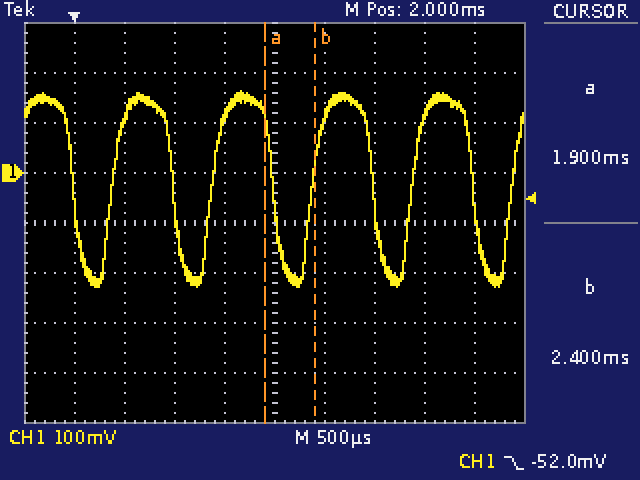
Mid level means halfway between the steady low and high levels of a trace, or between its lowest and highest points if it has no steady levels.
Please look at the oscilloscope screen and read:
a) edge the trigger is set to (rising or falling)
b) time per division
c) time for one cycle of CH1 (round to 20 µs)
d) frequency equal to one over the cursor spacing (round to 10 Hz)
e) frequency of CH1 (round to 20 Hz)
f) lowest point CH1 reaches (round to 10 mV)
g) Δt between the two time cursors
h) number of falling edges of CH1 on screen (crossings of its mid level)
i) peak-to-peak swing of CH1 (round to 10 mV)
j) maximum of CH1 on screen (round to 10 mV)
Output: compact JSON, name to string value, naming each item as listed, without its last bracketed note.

{"edge the trigger is set to": "falling", "time per division": "500 µs", "time for one cycle of CH1": "1.00 ms", "frequency equal to one over the cursor spacing": "2.00 kHz", "frequency of CH1": "1.00 kHz", "lowest point CH1 reaches": "-230 mV", "Δt between the two time cursors": "500 µs", "number of falling edges of CH1 on screen": "5", "peak-to-peak swing of CH1": "390 mV", "maximum of CH1 on screen": "160 mV"}
